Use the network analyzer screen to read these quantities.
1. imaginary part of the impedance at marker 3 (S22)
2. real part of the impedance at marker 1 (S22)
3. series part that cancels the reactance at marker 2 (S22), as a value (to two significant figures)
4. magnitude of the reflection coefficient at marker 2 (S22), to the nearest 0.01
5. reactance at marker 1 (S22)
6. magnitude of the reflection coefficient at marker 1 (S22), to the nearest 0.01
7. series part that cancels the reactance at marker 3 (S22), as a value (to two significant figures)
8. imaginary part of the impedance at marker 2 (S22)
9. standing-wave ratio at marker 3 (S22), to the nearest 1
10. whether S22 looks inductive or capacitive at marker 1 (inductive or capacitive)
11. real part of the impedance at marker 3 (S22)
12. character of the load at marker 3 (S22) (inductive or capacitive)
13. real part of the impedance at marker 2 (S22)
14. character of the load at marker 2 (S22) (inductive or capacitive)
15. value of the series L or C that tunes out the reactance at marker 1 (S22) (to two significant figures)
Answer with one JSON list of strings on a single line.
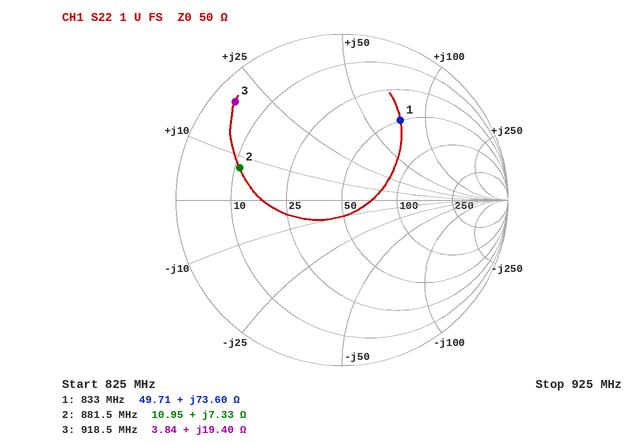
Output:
["+19.40 Ω", "49.71 Ω", "25 pF", "0.65", "+73.60 Ω", "0.59", "8.9 pF", "+7.33 Ω", "15", "inductive", "3.84 Ω", "inductive", "10.95 Ω", "inductive", "2.6 pF"]
